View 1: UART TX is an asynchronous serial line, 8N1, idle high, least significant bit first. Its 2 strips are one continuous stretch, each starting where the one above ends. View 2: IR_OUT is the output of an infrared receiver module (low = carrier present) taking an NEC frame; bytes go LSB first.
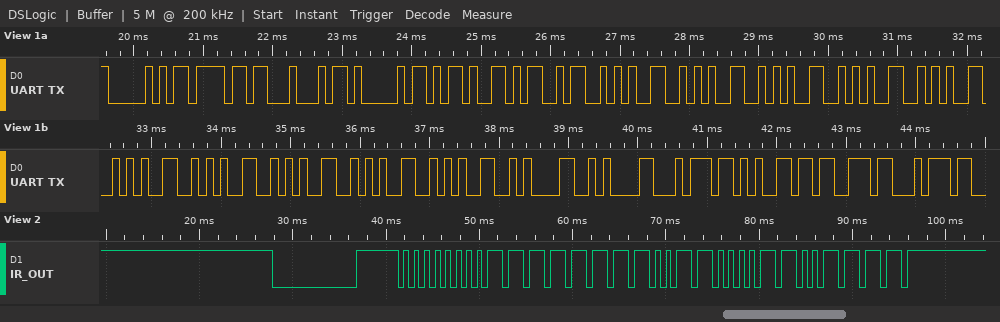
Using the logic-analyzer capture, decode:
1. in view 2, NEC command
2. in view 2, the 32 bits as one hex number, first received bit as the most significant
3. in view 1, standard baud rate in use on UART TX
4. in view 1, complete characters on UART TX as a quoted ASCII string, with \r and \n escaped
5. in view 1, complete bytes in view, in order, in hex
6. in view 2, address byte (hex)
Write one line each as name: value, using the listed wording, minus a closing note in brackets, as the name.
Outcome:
in view 2, NEC command: 0x0C
in view 2, the 32 bits as one hex number, first received bit as the most significant: 0x00FF30CF
in view 1, standard baud rate in use on UART TX: 9600 baud
in view 1, complete characters on UART TX as a quoted ASCII string, with \r and \n escaped: "PoDA-M**********\n\ntest"
in view 1, complete bytes in view, in order, in hex: 0x50 0x6F 0x44 0x41 0x2D 0x4D 0x2A 0x2A 0x2A 0x2A 0x2A 0x2A 0x2A 0x2A 0x2A 0x2A 0x0A 0x0A 0x74 0x65 0x73 0x74
in view 2, address byte: 0x00
